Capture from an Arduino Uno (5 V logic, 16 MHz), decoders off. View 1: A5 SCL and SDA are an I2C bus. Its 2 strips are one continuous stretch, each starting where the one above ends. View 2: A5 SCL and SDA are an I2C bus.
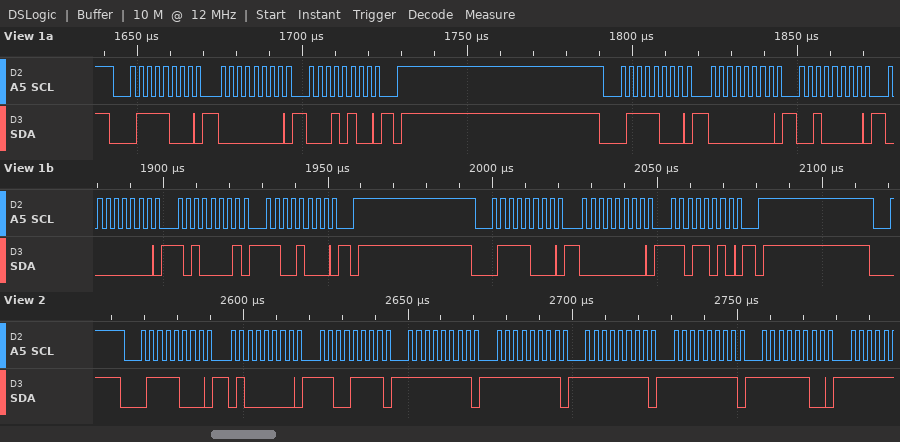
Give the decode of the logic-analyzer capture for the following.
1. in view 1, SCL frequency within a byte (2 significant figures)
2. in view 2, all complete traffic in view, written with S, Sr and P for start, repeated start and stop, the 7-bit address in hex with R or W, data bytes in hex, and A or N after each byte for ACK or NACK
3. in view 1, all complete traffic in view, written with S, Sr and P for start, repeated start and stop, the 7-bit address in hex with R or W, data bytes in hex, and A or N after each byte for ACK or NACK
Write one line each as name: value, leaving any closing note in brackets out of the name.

in view 1, SCL frequency within a byte: 400 kHz
in view 2, all complete traffic in view, written with S, Sr and P for start, repeated start and stop, the 7-bit address in hex with R or W, data bytes in hex, and A or N after each byte for ACK or NACK: S 3CW A 40 A CF A FF A FF A FF A FF A FC A
in view 1, all complete traffic in view, written with S, Sr and P for start, repeated start and stop, the 7-bit address in hex with R or W, data bytes in hex, and A or N after each byte for ACK or NACK: S 3CW A 00 A 14 A P S 3CW A 00 A 20 A 00 A A1 A C8 A P S 3CW A 00 A DA A P
